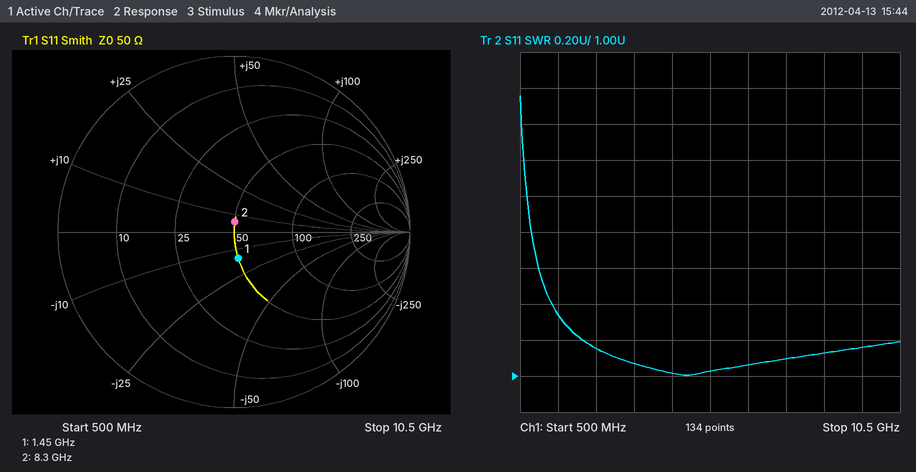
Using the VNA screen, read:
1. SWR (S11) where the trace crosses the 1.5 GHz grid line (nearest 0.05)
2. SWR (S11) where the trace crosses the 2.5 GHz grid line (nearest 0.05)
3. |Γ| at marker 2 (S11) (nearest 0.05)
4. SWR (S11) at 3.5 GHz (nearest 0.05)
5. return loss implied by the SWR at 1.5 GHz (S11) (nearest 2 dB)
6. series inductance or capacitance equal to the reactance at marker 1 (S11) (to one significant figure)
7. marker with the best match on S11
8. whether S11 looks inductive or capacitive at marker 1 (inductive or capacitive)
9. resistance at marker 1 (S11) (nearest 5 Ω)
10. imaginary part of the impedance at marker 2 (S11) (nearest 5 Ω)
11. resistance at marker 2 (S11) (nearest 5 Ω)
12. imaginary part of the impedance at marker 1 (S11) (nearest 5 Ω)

1.35
1.15
0.05
1.05
16 dB
7 pF
marker 2
capacitive
50 Ω
+5 Ω
50 Ω
-15 Ω
